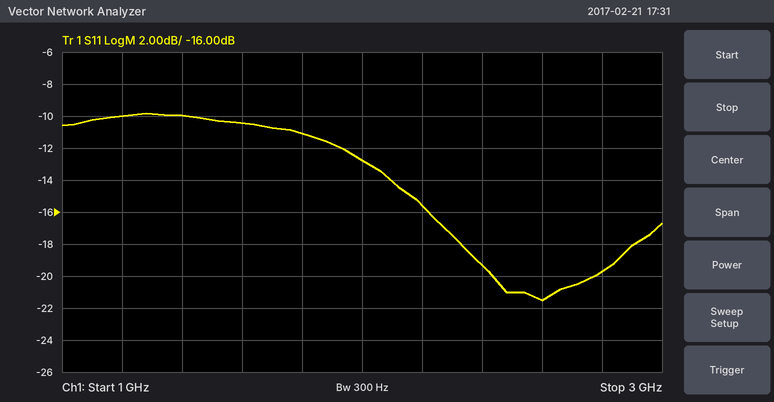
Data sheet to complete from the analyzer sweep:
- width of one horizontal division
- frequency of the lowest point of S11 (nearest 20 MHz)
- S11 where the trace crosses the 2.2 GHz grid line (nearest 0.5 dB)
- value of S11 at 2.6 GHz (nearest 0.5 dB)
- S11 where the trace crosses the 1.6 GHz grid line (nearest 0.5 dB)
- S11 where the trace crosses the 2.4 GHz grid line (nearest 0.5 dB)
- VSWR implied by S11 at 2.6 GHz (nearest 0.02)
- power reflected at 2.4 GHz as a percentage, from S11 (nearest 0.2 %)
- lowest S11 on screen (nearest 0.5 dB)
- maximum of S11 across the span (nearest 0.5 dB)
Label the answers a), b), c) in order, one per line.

a) 200 MHz
b) 2.60 GHz
c) -15.5 dB
d) -21.5 dB
e) -10.5 dB
f) -19.5 dB
g) 1.18
h) 1.2 %
i) -21.5 dB
j) -10.0 dB
